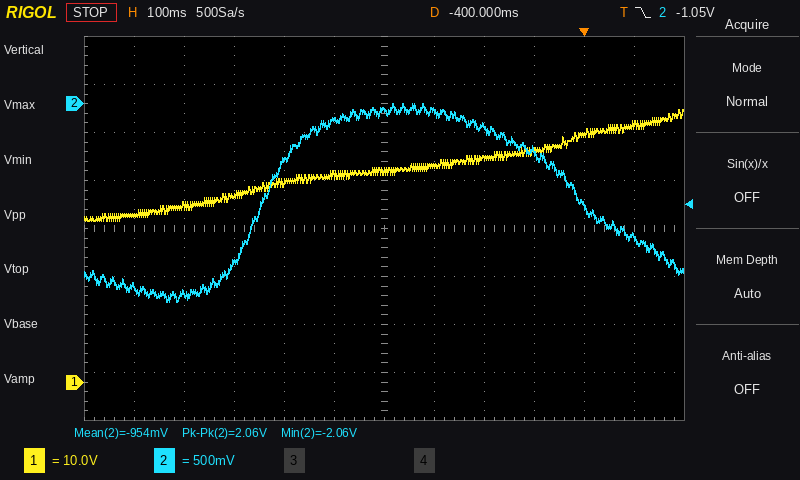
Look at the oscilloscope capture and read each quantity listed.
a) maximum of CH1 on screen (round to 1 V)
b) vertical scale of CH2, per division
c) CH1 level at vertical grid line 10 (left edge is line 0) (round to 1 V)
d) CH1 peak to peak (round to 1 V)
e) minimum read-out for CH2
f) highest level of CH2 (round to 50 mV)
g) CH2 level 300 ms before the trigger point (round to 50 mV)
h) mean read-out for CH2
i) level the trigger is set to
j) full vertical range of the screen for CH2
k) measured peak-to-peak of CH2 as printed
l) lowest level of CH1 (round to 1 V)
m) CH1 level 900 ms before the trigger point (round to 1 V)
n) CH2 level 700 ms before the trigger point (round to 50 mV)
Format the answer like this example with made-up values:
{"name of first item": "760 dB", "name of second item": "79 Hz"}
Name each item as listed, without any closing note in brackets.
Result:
{"maximum of CH1 on screen": "57 V", "vertical scale of CH2, per division": "500 mV", "CH1 level at vertical grid line 10 (left edge is line 0)": "52 V", "CH1 peak to peak": "23 V", "minimum read-out for CH2": "-2.06 V", "highest level of CH2": "0 mV", "CH2 level 300 ms before the trigger point": "-100 mV", "mean read-out for CH2": "-954 mV", "level the trigger is set to": "-1.05 V", "full vertical range of the screen for CH2": "4 V", "measured peak-to-peak of CH2 as printed": "2.06 V", "lowest level of CH1": "34 V", "CH1 level 900 ms before the trigger point": "35 V", "CH2 level 700 ms before the trigger point": "-1.65 V"}
